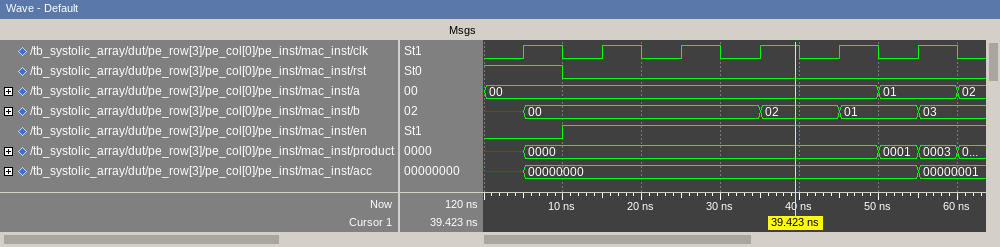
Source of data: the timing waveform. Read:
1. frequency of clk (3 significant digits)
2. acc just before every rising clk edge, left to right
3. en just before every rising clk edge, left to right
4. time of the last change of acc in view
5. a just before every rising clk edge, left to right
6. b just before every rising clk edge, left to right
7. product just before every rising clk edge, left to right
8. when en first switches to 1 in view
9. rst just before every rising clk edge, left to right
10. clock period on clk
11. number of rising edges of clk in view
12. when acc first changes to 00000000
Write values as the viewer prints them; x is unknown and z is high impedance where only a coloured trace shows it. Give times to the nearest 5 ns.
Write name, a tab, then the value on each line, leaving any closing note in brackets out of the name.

frequency of clk	100 MHz
acc just before every rising clk edge, left to right	x, 00000000, 00000000, 00000000, 00000000, 00000000
en just before every rising clk edge, left to right	0 1 1 1 1 1
time of the last change of acc in view	55 ns
a just before every rising clk edge, left to right	00, 00, 00, 00, 00, 01
b just before every rising clk edge, left to right	x, 00, 00, 00, 02, 01
product just before every rising clk edge, left to right	x, 0000, 0000, 0000, 0000, 0001
when en first switches to 1 in view	10 ns
rst just before every rising clk edge, left to right	1 0 0 0 0 0
clock period on clk	10 ns
number of rising edges of clk in view	6
when acc first changes to 00000000	5 ns
